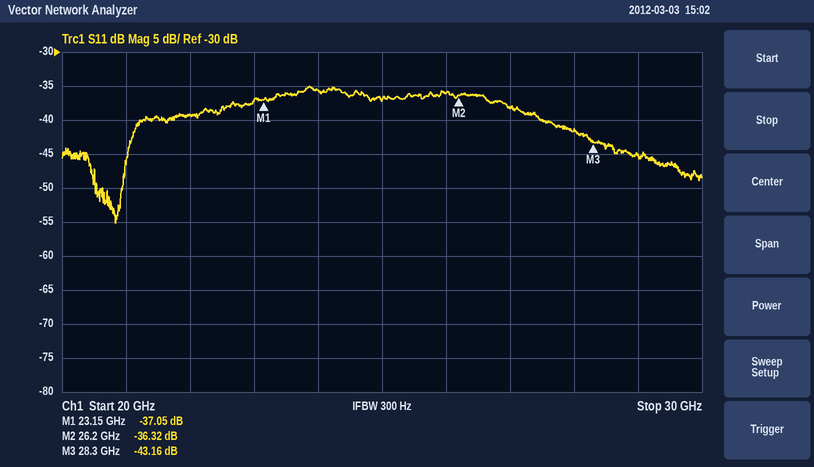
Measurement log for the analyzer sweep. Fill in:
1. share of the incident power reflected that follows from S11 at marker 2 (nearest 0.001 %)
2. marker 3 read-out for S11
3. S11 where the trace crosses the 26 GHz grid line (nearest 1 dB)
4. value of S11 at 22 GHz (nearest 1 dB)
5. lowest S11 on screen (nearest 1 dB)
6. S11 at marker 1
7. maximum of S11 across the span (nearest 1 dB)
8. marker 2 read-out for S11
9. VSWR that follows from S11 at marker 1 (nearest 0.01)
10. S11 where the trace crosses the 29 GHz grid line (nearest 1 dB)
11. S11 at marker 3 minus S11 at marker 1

0.023 %
-43.16 dB
-36 dB
-39 dB
-55 dB
-37.05 dB
-35 dB
-36.32 dB
1.03
-45 dB
-6.11 dB
